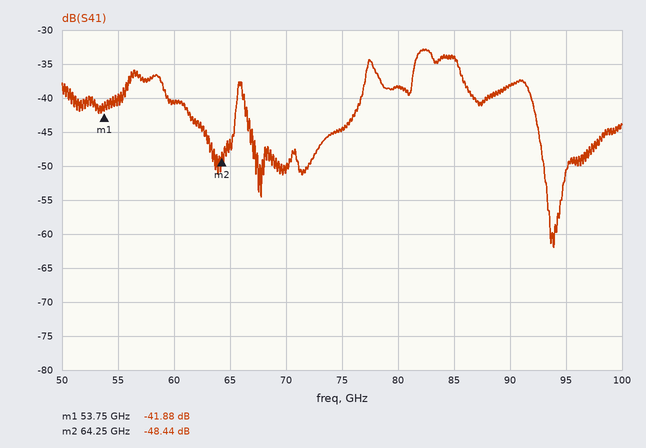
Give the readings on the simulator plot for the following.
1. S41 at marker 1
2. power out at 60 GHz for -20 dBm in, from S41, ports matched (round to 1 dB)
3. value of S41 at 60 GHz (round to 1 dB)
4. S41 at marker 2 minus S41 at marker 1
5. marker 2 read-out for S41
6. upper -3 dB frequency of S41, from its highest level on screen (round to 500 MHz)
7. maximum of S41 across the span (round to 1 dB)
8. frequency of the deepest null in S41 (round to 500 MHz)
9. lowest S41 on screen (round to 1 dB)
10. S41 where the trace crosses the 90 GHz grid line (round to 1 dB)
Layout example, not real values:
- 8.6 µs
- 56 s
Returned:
- -41.88 dB
- -61 dBm
- -41 dB
- -6.56 dB
- -48.44 dB
- 85.5 GHz
- -33 dB
- 94.0 GHz
- -62 dB
- -38 dB
